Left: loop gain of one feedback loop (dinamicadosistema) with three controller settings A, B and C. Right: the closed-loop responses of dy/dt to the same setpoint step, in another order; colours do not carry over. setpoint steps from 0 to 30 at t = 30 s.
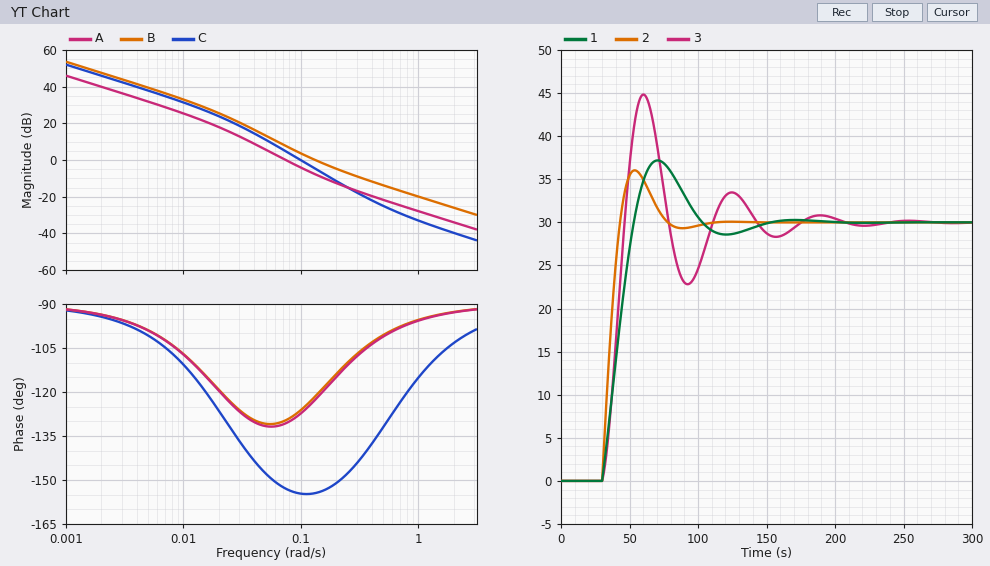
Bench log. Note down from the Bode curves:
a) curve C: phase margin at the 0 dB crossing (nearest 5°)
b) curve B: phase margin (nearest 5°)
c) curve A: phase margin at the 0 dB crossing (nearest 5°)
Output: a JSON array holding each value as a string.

["25°", "60°", "50°"]
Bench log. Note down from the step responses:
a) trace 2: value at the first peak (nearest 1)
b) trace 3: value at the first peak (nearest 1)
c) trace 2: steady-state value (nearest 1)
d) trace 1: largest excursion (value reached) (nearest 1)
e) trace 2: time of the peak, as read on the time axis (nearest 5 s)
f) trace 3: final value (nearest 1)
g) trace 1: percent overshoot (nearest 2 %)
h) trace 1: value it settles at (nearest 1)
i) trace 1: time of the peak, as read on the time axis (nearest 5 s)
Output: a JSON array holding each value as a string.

["36", "45", "30", "37", "55 s", "30", "24 %", "30", "70 s"]
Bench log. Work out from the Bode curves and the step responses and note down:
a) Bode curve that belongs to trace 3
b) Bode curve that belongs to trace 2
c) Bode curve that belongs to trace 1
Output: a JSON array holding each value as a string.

["C", "B", "A"]
